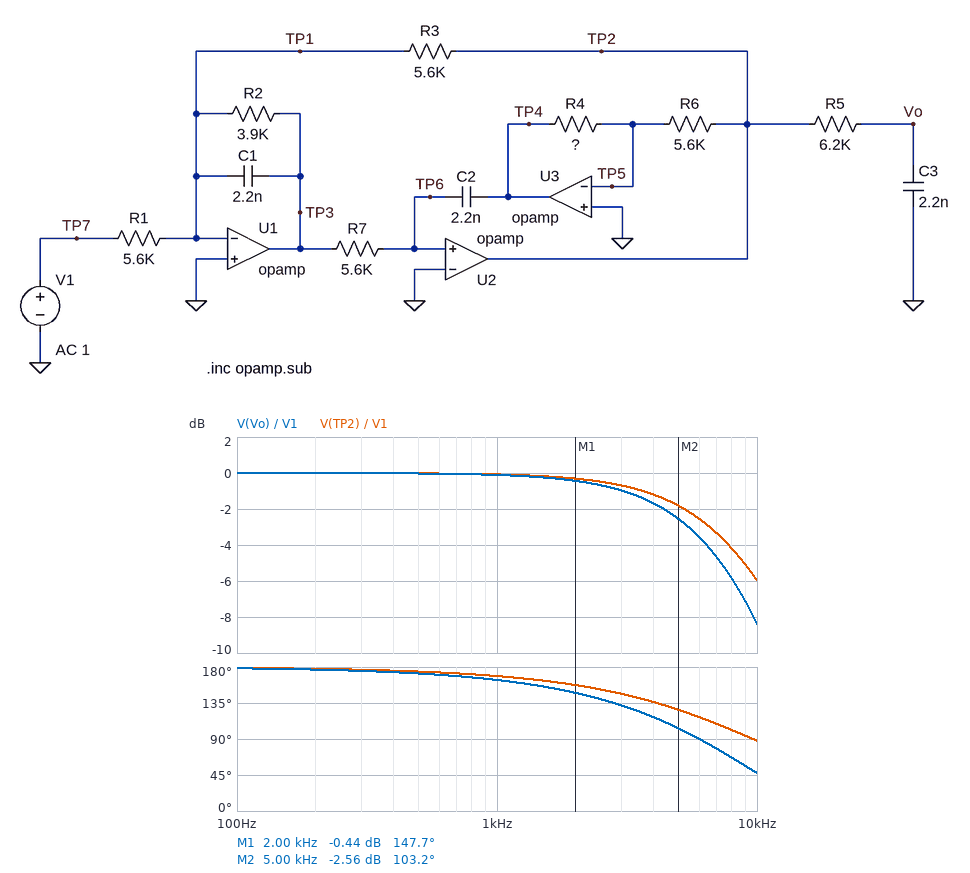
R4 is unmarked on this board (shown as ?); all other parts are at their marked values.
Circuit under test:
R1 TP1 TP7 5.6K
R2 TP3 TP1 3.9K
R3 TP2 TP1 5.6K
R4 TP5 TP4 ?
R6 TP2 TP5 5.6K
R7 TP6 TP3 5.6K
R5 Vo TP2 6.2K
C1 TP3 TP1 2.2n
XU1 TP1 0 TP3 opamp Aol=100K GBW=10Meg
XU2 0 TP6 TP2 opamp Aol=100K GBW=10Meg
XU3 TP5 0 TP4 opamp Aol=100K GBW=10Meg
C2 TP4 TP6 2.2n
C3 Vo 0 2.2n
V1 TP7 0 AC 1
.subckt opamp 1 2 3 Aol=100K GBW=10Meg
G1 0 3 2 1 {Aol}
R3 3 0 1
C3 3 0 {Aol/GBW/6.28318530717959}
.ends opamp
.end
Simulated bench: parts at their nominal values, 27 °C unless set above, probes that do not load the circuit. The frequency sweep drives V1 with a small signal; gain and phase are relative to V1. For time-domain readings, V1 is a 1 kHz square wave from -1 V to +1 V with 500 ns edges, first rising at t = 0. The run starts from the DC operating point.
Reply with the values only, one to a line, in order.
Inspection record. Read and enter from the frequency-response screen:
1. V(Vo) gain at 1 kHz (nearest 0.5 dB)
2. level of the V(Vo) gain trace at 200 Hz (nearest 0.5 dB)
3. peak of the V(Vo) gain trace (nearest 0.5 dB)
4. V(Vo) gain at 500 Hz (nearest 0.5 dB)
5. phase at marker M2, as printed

0 dB
0 dB
0 dB
0 dB
103.2 deg
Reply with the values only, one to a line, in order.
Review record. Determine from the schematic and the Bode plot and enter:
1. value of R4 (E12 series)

10 kΩ
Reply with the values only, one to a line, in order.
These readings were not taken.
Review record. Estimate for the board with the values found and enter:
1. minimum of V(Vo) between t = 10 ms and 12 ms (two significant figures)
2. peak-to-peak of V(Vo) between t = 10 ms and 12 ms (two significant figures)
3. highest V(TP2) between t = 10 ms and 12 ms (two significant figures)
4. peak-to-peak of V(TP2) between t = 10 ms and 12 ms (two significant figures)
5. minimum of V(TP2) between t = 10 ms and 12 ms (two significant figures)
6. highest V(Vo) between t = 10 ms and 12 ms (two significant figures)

-1.0 V
2.0 V
1.0 V
2.0 V
-1.0 V
1.0 V
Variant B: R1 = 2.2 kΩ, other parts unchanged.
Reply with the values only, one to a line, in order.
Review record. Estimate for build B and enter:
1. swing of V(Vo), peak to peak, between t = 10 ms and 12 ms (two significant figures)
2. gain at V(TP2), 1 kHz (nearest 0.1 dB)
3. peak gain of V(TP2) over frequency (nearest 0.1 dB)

5.1 V
8.0 dB
8.1 dB
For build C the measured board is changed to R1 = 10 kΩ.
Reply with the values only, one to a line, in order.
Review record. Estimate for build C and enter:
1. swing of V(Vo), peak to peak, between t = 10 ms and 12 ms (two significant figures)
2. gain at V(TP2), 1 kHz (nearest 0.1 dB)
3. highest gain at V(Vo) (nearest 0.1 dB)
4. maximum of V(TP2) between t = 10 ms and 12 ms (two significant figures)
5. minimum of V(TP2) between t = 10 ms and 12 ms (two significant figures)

1.1 V
-5.1 dB
-5.0 dB
560 mV
-560 mV
